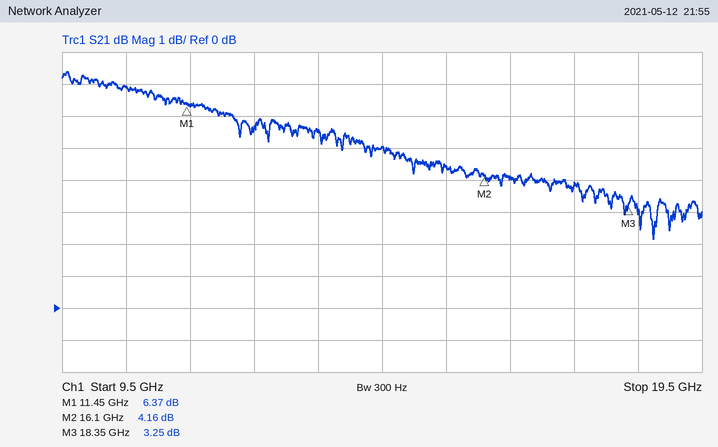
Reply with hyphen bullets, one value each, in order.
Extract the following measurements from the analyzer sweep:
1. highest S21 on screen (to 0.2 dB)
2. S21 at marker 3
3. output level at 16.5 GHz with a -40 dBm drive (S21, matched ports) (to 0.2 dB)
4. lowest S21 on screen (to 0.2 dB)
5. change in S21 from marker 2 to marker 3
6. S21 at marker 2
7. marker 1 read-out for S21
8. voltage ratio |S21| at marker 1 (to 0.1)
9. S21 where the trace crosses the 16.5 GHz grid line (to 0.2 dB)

- 7.4 dB
- 3.25 dB
- -36.0 dBm
- 2.2 dB
- -0.91 dB
- 4.16 dB
- 6.37 dB
- 2.1
- 4.0 dB
